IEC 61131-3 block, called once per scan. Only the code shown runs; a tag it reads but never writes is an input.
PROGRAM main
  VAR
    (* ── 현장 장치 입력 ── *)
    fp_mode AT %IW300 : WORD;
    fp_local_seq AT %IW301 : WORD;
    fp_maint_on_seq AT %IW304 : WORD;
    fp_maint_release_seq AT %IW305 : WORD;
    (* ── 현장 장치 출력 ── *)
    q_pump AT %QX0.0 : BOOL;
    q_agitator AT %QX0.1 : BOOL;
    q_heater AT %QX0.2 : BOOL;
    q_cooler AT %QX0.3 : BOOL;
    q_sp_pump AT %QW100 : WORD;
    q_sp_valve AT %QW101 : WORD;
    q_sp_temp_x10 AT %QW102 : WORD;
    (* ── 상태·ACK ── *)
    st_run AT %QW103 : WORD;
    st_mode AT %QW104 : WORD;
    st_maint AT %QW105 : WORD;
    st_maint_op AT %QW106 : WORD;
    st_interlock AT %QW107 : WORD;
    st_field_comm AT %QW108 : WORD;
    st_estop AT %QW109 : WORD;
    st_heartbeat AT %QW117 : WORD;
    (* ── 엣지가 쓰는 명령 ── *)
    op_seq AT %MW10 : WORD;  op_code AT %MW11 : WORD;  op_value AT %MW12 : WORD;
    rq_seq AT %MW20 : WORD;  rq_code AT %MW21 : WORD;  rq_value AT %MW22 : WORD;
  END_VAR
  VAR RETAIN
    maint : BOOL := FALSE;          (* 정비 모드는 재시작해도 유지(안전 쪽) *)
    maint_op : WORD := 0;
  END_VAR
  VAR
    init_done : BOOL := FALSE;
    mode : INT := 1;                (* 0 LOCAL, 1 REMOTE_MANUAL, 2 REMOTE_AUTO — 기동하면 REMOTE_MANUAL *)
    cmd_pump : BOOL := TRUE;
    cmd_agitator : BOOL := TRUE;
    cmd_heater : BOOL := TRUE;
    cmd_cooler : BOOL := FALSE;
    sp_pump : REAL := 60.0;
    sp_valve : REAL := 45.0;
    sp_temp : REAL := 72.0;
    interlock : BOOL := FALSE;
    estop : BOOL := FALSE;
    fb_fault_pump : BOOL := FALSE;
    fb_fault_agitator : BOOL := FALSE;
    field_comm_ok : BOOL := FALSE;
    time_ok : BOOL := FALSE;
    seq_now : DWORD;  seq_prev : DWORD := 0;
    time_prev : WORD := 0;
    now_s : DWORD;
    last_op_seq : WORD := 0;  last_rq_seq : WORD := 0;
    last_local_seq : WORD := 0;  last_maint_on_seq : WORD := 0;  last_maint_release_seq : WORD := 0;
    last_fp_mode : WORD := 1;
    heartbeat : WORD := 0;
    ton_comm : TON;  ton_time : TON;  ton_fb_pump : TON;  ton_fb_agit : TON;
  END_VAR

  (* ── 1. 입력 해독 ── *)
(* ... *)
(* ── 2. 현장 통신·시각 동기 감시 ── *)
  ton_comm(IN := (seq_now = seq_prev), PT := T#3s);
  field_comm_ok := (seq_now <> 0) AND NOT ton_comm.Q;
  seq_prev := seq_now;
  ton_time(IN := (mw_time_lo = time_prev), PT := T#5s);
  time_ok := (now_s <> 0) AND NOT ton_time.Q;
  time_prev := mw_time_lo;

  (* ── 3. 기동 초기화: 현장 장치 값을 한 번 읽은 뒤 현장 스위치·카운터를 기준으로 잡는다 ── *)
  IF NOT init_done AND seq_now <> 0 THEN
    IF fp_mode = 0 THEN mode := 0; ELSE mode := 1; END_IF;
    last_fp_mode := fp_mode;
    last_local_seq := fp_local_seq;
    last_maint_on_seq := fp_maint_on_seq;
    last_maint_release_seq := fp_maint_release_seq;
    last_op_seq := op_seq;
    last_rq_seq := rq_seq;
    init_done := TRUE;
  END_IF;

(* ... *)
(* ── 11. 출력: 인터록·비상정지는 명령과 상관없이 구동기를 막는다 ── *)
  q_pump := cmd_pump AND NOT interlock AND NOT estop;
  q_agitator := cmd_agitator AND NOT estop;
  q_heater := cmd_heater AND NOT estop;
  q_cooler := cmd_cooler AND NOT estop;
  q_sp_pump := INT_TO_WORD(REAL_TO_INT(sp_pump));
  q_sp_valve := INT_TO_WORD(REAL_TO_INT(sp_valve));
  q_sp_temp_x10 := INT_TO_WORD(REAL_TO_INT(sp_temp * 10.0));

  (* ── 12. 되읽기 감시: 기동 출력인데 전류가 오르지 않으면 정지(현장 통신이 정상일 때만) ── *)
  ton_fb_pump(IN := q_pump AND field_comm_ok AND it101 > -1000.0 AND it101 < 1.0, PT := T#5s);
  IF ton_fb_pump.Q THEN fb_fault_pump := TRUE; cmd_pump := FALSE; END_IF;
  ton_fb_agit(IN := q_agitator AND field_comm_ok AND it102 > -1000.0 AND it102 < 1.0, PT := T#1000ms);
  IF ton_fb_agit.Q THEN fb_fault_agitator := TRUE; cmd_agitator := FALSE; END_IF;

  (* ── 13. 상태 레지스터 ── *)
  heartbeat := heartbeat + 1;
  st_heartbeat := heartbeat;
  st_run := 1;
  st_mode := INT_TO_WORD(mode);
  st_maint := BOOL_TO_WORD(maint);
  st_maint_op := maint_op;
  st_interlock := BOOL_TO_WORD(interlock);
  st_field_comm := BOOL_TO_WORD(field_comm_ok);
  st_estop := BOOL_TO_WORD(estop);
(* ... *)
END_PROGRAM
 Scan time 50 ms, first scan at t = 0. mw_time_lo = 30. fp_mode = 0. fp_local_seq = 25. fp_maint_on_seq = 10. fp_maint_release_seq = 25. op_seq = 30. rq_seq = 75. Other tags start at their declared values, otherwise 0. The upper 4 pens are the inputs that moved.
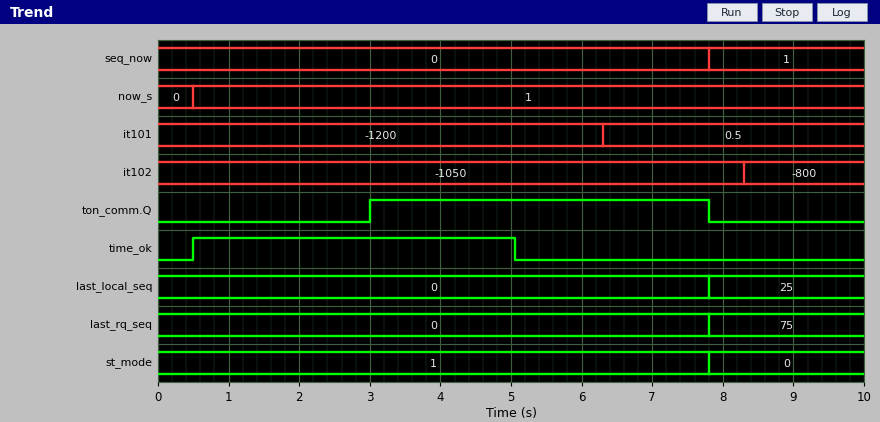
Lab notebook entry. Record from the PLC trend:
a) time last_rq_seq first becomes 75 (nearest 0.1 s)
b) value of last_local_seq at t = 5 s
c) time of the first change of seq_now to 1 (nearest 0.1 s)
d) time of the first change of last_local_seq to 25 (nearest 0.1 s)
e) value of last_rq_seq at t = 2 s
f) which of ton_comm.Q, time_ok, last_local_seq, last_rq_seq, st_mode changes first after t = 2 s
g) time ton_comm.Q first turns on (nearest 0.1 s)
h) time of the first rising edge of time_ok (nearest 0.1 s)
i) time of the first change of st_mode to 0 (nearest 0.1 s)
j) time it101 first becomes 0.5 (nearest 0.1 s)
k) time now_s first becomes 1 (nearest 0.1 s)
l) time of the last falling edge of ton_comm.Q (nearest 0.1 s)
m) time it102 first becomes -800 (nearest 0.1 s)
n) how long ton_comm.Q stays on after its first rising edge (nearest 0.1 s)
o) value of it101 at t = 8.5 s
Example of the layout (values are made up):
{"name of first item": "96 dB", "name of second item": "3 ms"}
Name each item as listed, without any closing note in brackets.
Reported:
{"time last_rq_seq first becomes 75": "7.8 s", "value of last_local_seq at t = 5 s": "0", "time of the first change of seq_now to 1": "7.8 s", "time of the first change of last_local_seq to 25": "7.8 s", "value of last_rq_seq at t = 2 s": "0", "which of ton_comm.Q, time_ok, last_local_seq, last_rq_seq, st_mode changes first after t = 2 s": "ton_comm.Q", "time ton_comm.Q first turns on": "3.0 s", "time of the first rising edge of time_ok": "0.5 s", "time of the first change of st_mode to 0": "7.8 s", "time it101 first becomes 0.5": "6.3 s", "time now_s first becomes 1": "0.5 s", "time of the last falling edge of ton_comm.Q": "7.8 s", "time it102 first becomes -800": "8.3 s", "how long ton_comm.Q stays on after its first rising edge": "4.8 s", "value of it101 at t = 8.5 s": "0.5"}
